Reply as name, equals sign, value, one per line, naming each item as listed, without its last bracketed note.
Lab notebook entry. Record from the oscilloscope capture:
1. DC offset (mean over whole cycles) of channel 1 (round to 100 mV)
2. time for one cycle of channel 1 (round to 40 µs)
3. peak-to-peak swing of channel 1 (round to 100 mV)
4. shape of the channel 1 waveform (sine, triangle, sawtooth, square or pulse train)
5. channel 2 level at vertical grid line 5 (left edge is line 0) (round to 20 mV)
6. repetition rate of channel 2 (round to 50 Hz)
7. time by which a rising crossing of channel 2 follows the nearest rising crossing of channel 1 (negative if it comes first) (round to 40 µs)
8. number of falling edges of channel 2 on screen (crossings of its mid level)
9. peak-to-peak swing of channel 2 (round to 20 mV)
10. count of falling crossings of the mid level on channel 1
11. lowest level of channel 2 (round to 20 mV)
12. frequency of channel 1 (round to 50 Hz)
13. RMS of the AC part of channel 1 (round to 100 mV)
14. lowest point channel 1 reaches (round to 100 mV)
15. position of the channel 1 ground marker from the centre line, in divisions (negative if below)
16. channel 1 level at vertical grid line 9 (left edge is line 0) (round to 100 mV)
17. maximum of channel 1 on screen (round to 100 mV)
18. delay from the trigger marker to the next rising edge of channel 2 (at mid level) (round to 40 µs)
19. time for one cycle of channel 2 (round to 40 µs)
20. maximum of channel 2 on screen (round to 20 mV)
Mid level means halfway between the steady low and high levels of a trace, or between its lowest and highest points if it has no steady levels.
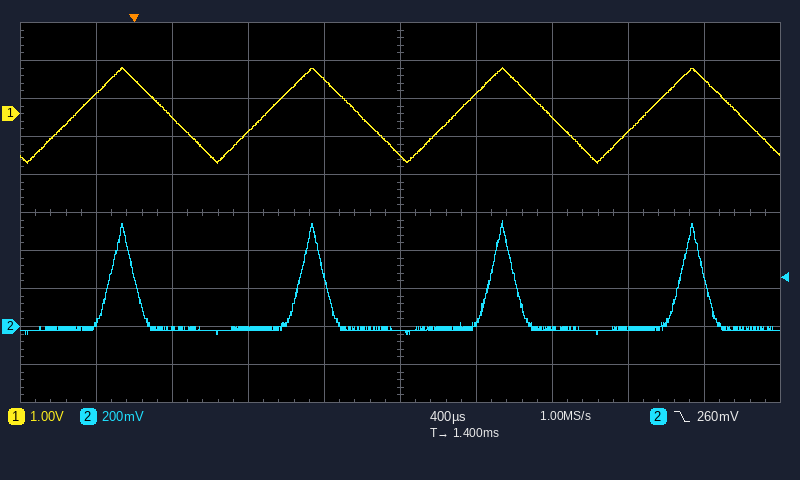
DC offset (mean over whole cycles) of channel 1 = 0.0 V
time for one cycle of channel 1 = 1.00 ms
peak-to-peak swing of channel 1 = 2.5 V
shape of the channel 1 waveform = triangle
channel 2 level at vertical grid line 5 (left edge is line 0) = -20 mV
repetition rate of channel 2 = 1.00 kHz
time by which a rising crossing of channel 2 follows the nearest rising crossing of channel 1 (negative if it comes first) = +200 µs
number of falling edges of channel 2 on screen = 4
peak-to-peak swing of channel 2 = 600 mV
count of falling crossings of the mid level on channel 1 = 4
lowest level of channel 2 = -40 mV
frequency of channel 1 = 1.00 kHz
RMS of the AC part of channel 1 = 700 mV
lowest point channel 1 reaches = -1.3 V
position of the channel 1 ground marker from the centre line, in divisions = +2.6 div
channel 1 level at vertical grid line 9 (left edge is line 0) = 900 mV
maximum of channel 1 on screen = 1.2 V
delay from the trigger marker to the next rising edge of channel 2 (at mid level) = 880 µs
time for one cycle of channel 2 = 1.00 ms
maximum of channel 2 on screen = 560 mV
